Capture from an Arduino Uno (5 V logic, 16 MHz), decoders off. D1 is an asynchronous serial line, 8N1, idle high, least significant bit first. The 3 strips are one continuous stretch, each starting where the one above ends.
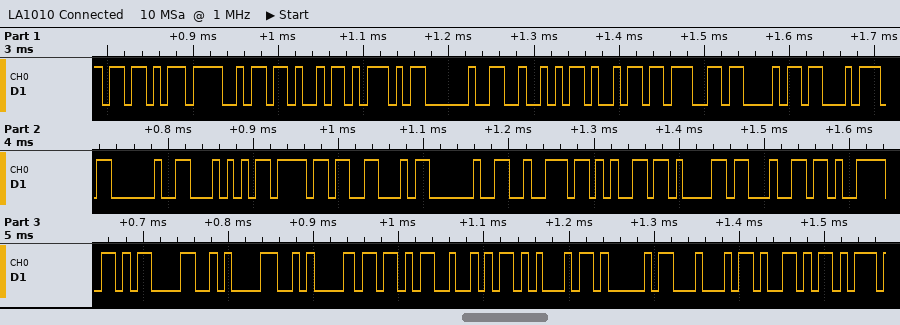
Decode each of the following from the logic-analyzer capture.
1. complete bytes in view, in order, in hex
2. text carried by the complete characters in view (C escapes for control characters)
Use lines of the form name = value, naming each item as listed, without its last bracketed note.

complete bytes in view, in order, in hex = 5B 4F 4B 5D 20 52 69 67 68 74 20 54 6F 46 20 72 65 61 64 79 0D 0A 0A 5B 52 45 41 44 59
text carried by the complete characters in view = "[OK] Right ToF ready\r\n\n[READY"
